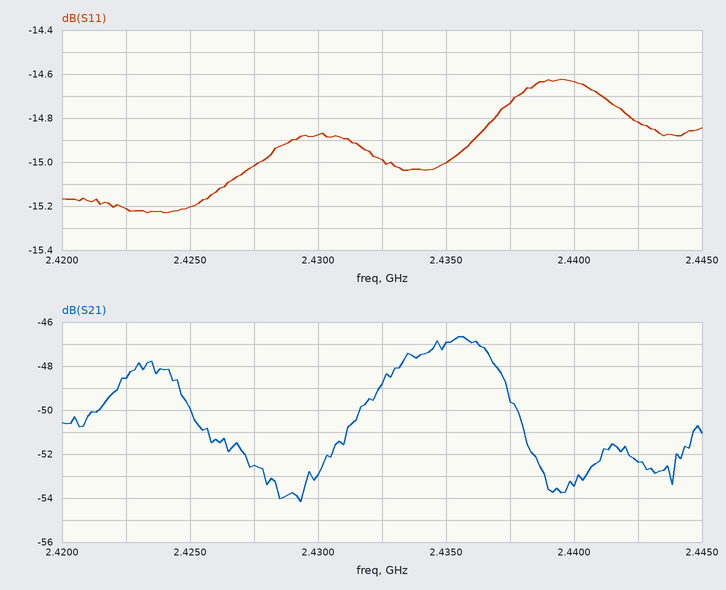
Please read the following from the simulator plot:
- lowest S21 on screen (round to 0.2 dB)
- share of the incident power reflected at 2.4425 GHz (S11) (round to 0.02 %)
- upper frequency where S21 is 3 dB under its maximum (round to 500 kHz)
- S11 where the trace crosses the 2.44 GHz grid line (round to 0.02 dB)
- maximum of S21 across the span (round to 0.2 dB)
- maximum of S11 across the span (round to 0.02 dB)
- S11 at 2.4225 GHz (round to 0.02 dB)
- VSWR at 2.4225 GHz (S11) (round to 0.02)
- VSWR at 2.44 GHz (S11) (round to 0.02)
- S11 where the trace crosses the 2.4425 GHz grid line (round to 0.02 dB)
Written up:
-54.2 dB
3.30 %
2.4375 GHz
-14.64 dB
-46.6 dB
-14.62 dB
-15.22 dB
1.42
1.46
-14.82 dB
